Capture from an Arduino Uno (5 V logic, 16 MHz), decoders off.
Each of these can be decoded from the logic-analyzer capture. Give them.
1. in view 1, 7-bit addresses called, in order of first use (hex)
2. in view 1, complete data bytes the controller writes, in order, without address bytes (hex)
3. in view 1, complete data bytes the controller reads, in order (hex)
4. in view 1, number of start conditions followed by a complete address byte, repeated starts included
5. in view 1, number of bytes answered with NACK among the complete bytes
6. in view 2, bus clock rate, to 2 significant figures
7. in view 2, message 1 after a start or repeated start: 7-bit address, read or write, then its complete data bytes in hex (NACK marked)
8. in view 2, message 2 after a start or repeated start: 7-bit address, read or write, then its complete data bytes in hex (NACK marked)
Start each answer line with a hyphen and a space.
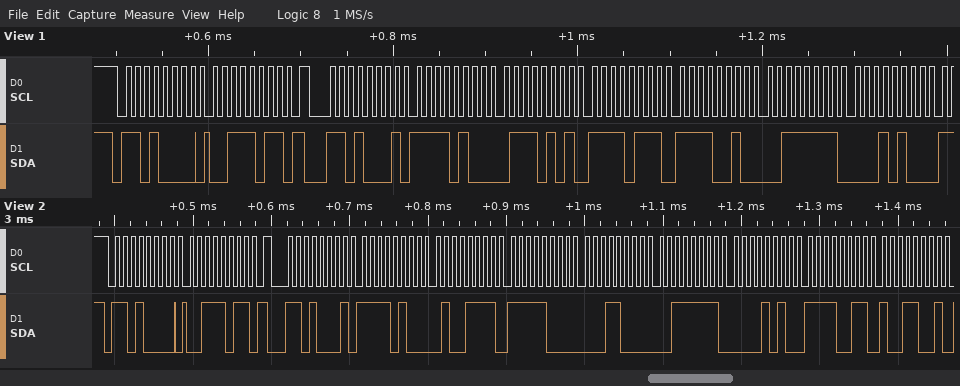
- 0x68
- 3B
- F4 75 F7 F2 3F 14
- 2
- 0
- 100 kHz
- 0x68 write: 3B
- 0x68 read: F4 4F F8 18 3F 0A F3 99
